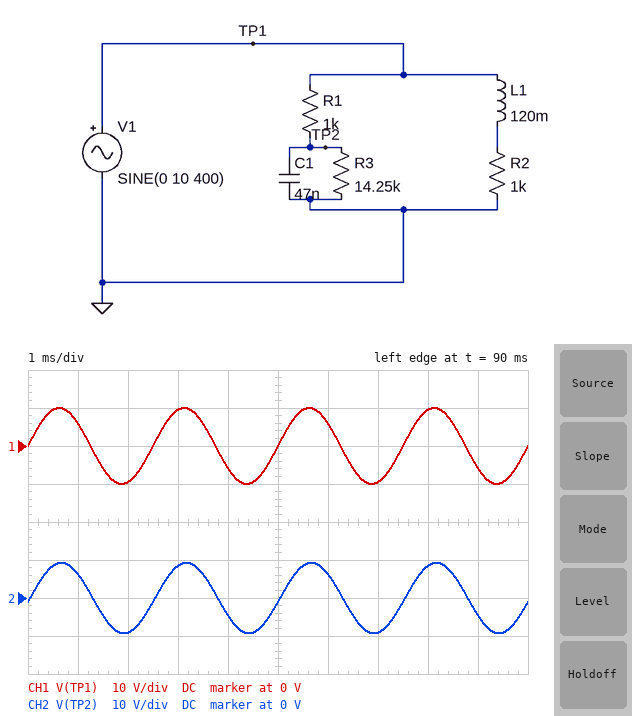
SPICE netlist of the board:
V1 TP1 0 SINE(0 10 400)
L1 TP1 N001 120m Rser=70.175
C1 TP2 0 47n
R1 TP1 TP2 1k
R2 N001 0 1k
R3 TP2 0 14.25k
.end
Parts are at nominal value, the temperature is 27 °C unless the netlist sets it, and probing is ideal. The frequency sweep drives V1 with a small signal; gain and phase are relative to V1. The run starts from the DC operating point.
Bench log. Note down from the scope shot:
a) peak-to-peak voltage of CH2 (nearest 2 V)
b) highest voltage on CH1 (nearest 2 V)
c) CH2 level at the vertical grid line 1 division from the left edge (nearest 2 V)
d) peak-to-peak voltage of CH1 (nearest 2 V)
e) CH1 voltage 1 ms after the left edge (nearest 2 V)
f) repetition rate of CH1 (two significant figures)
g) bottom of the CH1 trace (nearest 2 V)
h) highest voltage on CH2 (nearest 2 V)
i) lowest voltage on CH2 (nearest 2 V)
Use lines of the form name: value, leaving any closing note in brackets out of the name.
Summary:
peak-to-peak voltage of CH2: 18 V
highest voltage on CH1: 10 V
CH2 level at the vertical grid line 1 division from the left edge: 6 V
peak-to-peak voltage of CH1: 20 V
CH1 voltage 1 ms after the left edge: 6 V
repetition rate of CH1: 400 Hz
bottom of the CH1 trace: -10 V
highest voltage on CH2: 10 V
lowest voltage on CH2: -10 V
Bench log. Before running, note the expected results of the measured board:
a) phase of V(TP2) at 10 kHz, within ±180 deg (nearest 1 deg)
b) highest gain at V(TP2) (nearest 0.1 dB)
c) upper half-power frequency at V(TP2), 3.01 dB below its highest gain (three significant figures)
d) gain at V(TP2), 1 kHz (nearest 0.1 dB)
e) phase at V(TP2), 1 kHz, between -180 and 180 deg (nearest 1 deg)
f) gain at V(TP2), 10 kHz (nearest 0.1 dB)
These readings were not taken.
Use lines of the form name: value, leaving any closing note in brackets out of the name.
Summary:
phase of V(TP2) at 10 kHz, within ±180 deg: -70 deg
highest gain at V(TP2): -0.6 dB
upper half-power frequency at V(TP2), 3.01 dB below its highest gain: 3.62 kHz
gain at V(TP2), 1 kHz: -0.9 dB
phase at V(TP2), 1 kHz, between -180 and 180 deg: -15 deg
gain at V(TP2), 10 kHz: -9.9 dB
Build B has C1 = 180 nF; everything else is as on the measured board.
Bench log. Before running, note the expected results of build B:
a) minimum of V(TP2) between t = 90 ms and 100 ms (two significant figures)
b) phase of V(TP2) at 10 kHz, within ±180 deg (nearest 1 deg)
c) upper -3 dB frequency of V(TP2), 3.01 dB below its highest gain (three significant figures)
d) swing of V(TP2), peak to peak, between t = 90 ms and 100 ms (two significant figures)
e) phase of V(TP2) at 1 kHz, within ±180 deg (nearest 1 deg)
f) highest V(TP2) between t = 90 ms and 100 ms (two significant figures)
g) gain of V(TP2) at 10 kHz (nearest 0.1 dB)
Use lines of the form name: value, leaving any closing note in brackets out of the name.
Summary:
minimum of V(TP2) between t = 90 ms and 100 ms: -8.6 V
phase of V(TP2) at 10 kHz, within ±180 deg: -85 deg
upper -3 dB frequency of V(TP2), 3.01 dB below its highest gain: 946 Hz
swing of V(TP2), peak to peak, between t = 90 ms and 100 ms: 17 V
phase of V(TP2) at 1 kHz, within ±180 deg: -47 deg
highest V(TP2) between t = 90 ms and 100 ms: 8.6 V
gain of V(TP2) at 10 kHz: -21.1 dB
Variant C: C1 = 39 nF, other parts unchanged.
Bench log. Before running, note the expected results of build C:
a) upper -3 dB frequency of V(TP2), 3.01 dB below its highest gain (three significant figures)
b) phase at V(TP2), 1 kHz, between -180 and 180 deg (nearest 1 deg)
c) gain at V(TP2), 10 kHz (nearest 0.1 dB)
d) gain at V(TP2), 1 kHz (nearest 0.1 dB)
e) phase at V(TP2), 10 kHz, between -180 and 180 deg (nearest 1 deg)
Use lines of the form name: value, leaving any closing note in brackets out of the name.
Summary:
upper -3 dB frequency of V(TP2), 3.01 dB below its highest gain: 4.37 kHz
phase at V(TP2), 1 kHz, between -180 and 180 deg: -13 deg
gain at V(TP2), 10 kHz: -8.5 dB
gain at V(TP2), 1 kHz: -0.8 dB
phase at V(TP2), 10 kHz, between -180 and 180 deg: -66 deg
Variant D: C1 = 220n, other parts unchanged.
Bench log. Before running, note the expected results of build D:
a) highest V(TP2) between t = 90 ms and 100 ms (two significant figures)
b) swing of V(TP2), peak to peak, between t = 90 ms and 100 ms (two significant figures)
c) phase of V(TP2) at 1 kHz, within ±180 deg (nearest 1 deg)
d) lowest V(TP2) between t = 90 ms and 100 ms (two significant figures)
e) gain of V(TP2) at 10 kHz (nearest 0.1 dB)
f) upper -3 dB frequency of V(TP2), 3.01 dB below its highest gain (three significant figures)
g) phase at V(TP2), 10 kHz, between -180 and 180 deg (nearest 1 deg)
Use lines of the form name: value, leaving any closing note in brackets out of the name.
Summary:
highest V(TP2) between t = 90 ms and 100 ms: 8.3 V
swing of V(TP2), peak to peak, between t = 90 ms and 100 ms: 17 V
phase of V(TP2) at 1 kHz, within ±180 deg: -52 deg
lowest V(TP2) between t = 90 ms and 100 ms: -8.3 V
gain of V(TP2) at 10 kHz: -22.8 dB
upper -3 dB frequency of V(TP2), 3.01 dB below its highest gain: 774 Hz
phase at V(TP2), 10 kHz, between -180 and 180 deg: -86 deg
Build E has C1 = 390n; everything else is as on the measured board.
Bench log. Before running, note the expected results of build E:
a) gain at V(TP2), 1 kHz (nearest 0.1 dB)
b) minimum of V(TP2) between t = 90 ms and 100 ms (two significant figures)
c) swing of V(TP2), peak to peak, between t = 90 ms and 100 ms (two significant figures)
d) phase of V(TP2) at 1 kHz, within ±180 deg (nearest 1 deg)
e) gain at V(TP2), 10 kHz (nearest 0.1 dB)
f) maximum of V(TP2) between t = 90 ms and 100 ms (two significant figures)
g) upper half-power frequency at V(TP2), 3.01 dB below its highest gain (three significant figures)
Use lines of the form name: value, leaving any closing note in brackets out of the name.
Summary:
gain at V(TP2), 1 kHz: -8.5 dB
minimum of V(TP2) between t = 90 ms and 100 ms: -6.9 V
swing of V(TP2), peak to peak, between t = 90 ms and 100 ms: 14 V
phase of V(TP2) at 1 kHz, within ±180 deg: -66 deg
gain at V(TP2), 10 kHz: -27.8 dB
maximum of V(TP2) between t = 90 ms and 100 ms: 6.9 V
upper half-power frequency at V(TP2), 3.01 dB below its highest gain: 437 Hz
